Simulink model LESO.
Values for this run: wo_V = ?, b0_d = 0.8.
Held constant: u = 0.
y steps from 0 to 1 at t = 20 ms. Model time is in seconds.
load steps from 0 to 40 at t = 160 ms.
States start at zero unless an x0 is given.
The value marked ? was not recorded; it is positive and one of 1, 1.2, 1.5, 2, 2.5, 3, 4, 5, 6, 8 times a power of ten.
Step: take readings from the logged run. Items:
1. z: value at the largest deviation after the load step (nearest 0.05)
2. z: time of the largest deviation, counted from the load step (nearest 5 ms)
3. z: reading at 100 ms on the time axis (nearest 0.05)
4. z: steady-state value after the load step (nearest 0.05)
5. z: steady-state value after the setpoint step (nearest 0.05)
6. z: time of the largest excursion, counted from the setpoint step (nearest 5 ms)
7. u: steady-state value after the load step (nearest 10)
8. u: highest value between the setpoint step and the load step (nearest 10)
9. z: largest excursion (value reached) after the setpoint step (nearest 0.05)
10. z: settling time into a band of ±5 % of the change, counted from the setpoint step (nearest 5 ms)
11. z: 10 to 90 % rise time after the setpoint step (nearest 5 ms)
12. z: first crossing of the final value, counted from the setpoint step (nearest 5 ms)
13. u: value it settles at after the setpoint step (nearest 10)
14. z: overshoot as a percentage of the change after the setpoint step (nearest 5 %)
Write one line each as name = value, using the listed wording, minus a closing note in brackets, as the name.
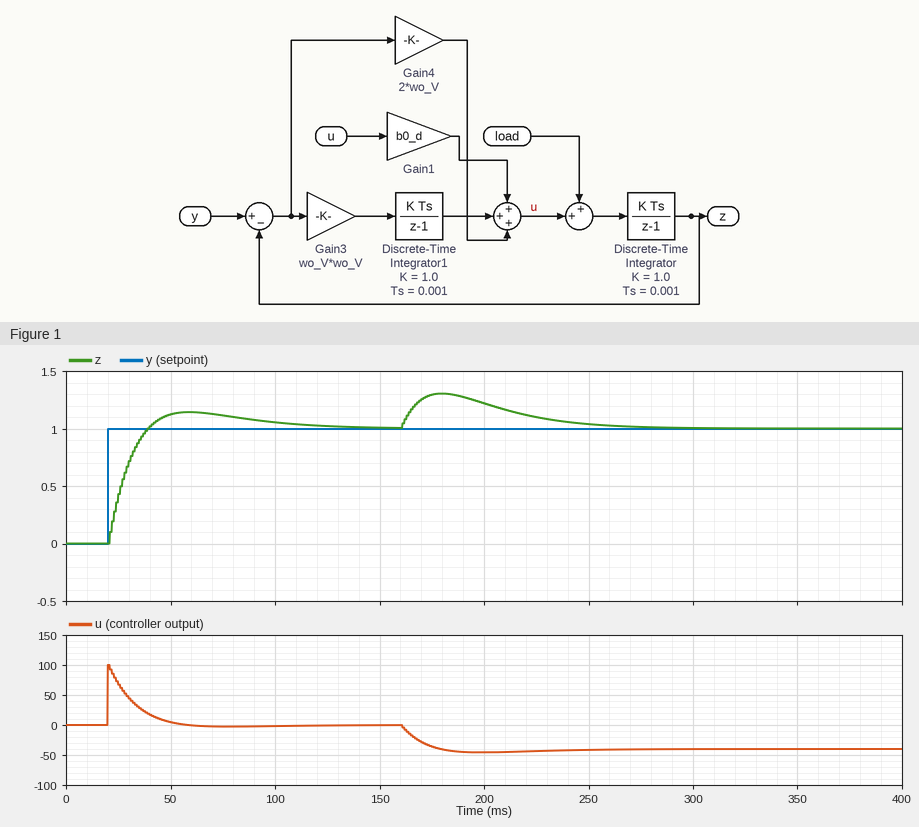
z: value at the largest deviation after the load step = 1.30
z: time of the largest deviation, counted from the load step = 20 ms
z: reading at 100 ms on the time axis = 1.05
z: steady-state value after the load step = 1.00
z: steady-state value after the setpoint step = 1.00
z: time of the largest excursion, counted from the setpoint step = 40 ms
u: steady-state value after the load step = -40
u: highest value between the setpoint step and the load step = 100
z: largest excursion (value reached) after the setpoint step = 1.15
z: settling time into a band of ±5 % of the change, counted from the setpoint step = 80 ms
z: 10 to 90 % rise time after the setpoint step = 15 ms
z: first crossing of the final value, counted from the setpoint step = 20 ms
u: value it settles at after the setpoint step = 0
z: overshoot as a percentage of the change after the setpoint step = 15 %
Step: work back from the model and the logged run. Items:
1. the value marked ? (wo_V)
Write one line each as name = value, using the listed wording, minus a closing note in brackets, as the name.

the value marked ? = 50
